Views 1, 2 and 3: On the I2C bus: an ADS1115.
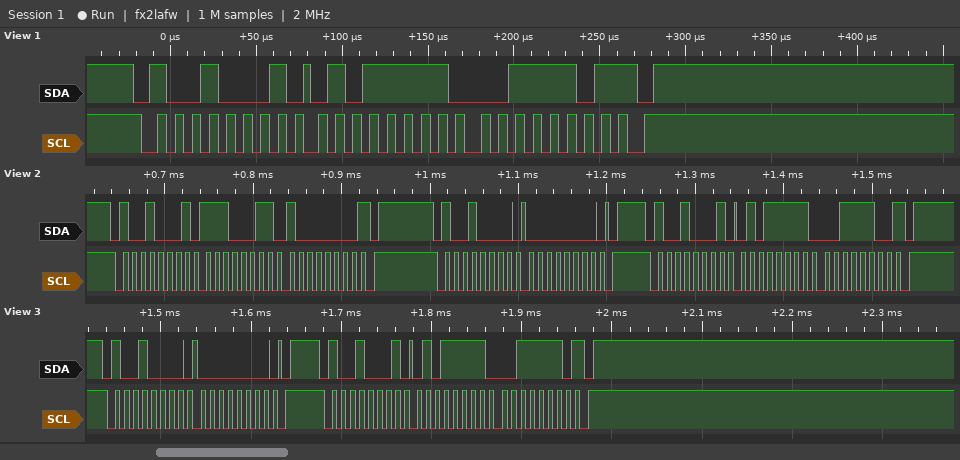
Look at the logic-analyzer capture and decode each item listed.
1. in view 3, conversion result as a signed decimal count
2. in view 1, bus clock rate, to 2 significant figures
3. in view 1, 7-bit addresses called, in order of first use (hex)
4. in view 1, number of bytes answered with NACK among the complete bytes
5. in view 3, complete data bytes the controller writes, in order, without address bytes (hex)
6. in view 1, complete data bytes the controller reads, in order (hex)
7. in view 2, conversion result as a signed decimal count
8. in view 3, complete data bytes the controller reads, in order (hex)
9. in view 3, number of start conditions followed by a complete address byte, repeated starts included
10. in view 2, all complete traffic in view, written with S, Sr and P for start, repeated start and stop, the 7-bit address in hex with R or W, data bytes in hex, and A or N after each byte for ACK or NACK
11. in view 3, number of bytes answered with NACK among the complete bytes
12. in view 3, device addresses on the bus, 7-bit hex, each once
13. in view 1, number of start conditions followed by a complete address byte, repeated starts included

24382
100 kHz
0x48
1
00
5F 3D
24380
5F 3E
2
S 48R A E3 A 80 N P S 48W A 00 A P S 48R A 5F A 3C N P
1
0x48
1
